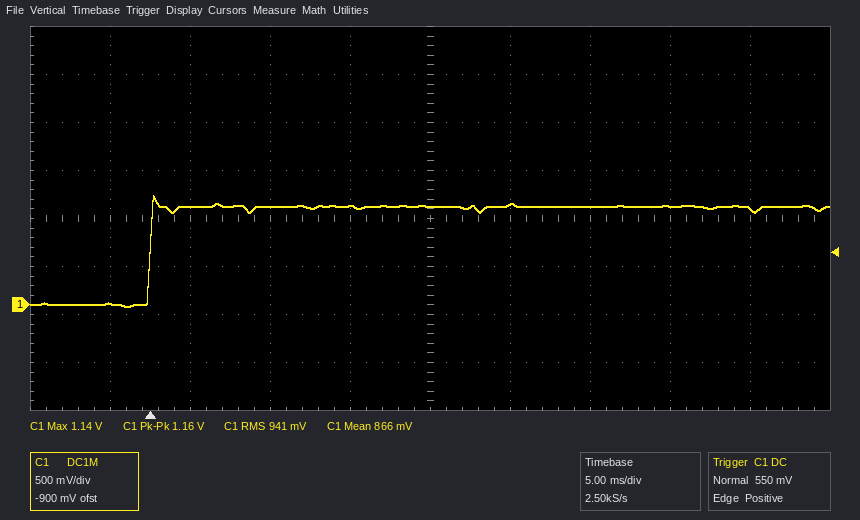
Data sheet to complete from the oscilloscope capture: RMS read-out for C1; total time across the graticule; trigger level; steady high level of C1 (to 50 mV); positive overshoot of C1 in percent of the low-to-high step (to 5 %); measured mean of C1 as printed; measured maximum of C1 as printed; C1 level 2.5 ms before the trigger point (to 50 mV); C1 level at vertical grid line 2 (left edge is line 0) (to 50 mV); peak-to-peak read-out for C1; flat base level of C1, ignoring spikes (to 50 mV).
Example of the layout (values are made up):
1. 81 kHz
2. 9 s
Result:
1. 941 mV
2. 50 ms
3. 550 mV
4. 1.00 V
5. 10 %
6. 866 mV
7. 1.14 V
8. 0 mV
9. 1.00 V
10. 1.16 V
11. 0 mV
